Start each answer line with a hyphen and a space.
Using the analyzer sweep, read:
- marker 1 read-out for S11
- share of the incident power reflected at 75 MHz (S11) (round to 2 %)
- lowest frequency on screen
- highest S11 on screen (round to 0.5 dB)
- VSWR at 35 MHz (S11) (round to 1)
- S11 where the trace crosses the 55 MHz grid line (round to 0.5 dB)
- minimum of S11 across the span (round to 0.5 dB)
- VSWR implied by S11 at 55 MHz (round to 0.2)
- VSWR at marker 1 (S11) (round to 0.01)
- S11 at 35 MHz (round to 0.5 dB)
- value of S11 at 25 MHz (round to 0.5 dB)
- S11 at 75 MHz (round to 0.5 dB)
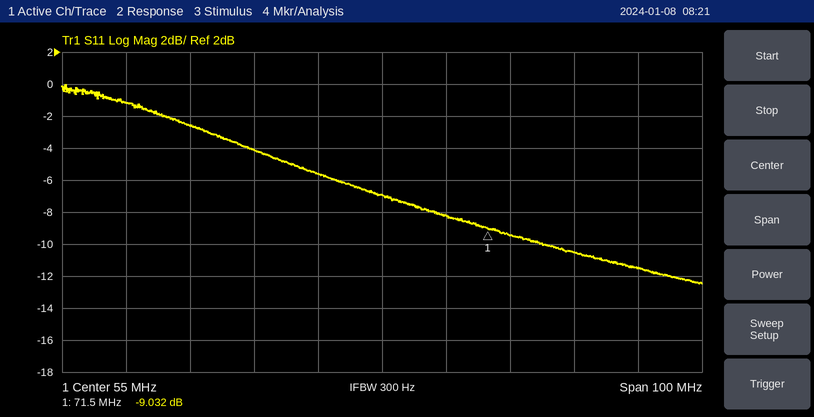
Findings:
- -9.032 dB
- 12 %
- 5 MHz
- 0.0 dB
- 4
- -7.0 dB
- -12.5 dB
- 2.6
- 2.09
- -4.0 dB
- -2.5 dB
- -9.5 dB
